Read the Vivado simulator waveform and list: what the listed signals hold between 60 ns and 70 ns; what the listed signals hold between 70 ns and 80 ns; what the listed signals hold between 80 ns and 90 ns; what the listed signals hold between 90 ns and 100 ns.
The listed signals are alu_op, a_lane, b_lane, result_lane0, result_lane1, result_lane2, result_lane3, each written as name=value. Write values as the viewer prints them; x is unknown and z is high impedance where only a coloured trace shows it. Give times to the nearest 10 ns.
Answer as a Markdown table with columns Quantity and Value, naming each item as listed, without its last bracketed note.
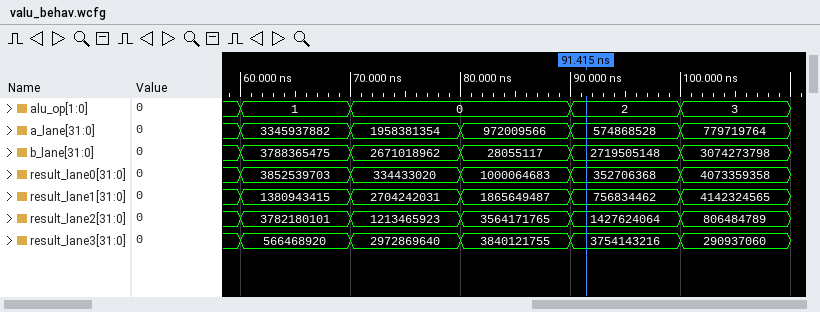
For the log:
| Quantity | Value |
|---|---|
| what the listed signals hold between 60 ns and 70 ns | alu_op=1, a_lane=3345937882, b_lane=3788365475, result_lane0=3852539703, result_lane1=1380943415, result_lane2=3782180101, result_lane3=566468920 |
| what the listed signals hold between 70 ns and 80 ns | alu_op=0, a_lane=1958381354, b_lane=2671018962, result_lane0=334433020, result_lane1=2704242031, result_lane2=1213465923, result_lane3=2972869640 |
| what the listed signals hold between 80 ns and 90 ns | alu_op=0, a_lane=972009566, b_lane=28055117, result_lane0=1000064683, result_lane1=1865649487, result_lane2=3564171765, result_lane3=3840121755 |
| what the listed signals hold between 90 ns and 100 ns | alu_op=2, a_lane=574868528, b_lane=2719505148, result_lane0=352706368, result_lane1=756834462, result_lane2=1427624064, result_lane3=3754143216 |
